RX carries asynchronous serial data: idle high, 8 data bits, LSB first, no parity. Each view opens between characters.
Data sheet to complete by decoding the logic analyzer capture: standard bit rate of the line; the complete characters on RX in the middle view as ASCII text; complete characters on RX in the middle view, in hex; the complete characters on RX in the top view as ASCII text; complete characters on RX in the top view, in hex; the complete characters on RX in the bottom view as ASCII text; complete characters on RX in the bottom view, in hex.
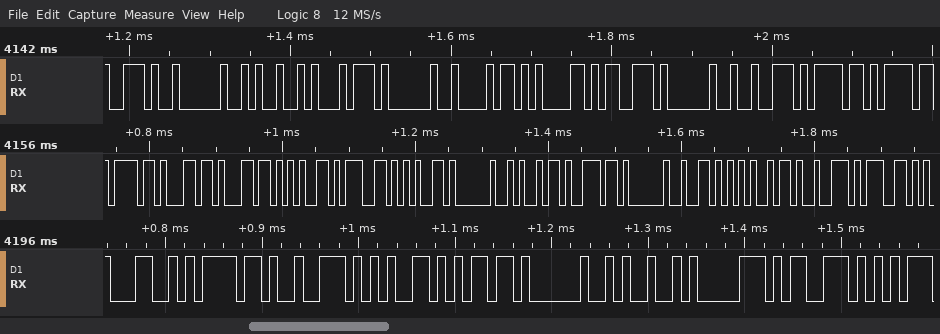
115200 baud
"ollege in Virg"
6F, 6C, 6C, 65, 67, 65, 20, 69, 6E, 20, 56, 69, 72, 67
". It has ro"
2E, 20, 49, 74, 20, 68, 61, 73, 20, 72, 6F
"Lorem Ips"
4C, 6F, 72, 65, 6D, 20, 49, 70, 73
